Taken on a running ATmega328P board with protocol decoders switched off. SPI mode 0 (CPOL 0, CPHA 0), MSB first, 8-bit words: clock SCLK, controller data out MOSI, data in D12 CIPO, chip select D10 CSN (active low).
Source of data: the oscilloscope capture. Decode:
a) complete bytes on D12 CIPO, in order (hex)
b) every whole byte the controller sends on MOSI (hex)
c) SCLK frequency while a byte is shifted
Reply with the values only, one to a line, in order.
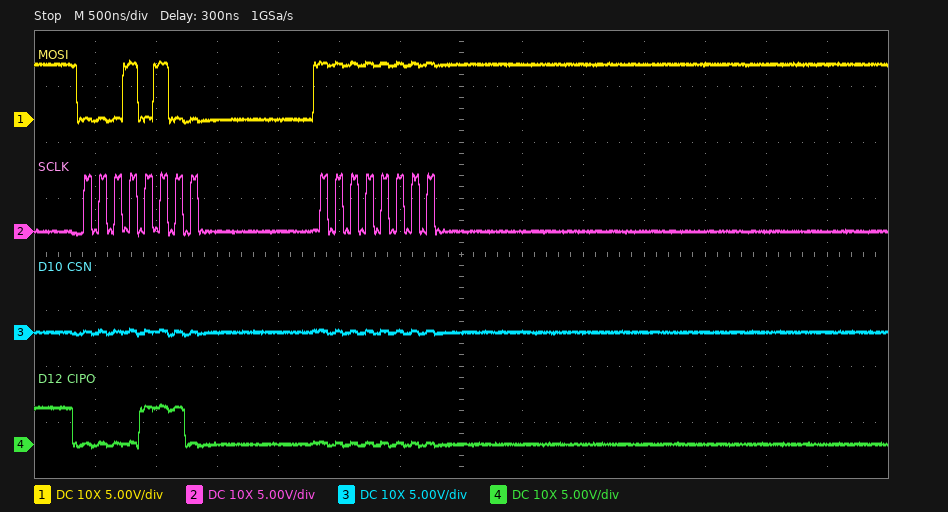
0E 00
14 FF
8 MHz
